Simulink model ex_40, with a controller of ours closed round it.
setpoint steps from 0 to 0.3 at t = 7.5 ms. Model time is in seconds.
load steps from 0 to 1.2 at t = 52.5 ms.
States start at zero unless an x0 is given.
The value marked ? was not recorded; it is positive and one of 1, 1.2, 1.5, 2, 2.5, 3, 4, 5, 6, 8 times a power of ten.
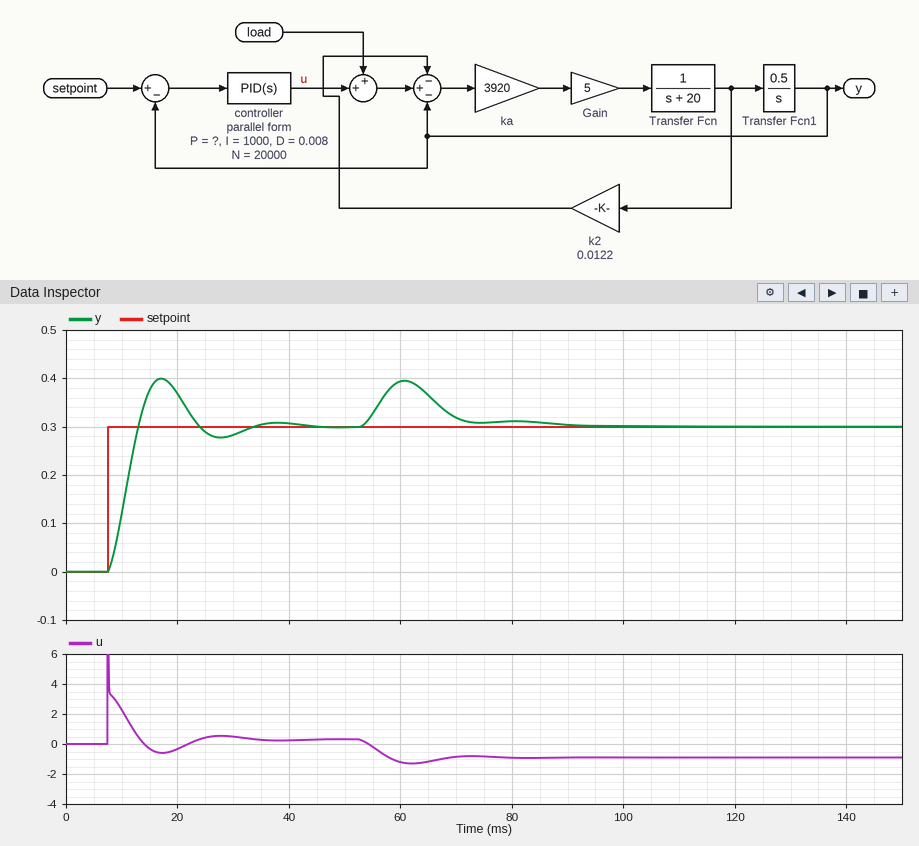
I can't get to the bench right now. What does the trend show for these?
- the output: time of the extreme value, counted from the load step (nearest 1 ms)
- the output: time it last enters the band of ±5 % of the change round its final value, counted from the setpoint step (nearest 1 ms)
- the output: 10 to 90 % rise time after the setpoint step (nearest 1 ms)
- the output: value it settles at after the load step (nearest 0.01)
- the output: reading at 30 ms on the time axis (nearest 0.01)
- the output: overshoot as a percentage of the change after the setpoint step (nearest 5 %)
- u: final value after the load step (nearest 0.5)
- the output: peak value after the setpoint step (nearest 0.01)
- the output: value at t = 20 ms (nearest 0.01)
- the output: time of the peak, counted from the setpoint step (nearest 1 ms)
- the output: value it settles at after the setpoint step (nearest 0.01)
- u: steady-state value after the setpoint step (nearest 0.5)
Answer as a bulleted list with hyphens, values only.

- 8 ms
- 23 ms
- 4 ms
- 0.30
- 0.28
- 35 %
- -1.0
- 0.40
- 0.37
- 10 ms
- 0.30
- 0.5
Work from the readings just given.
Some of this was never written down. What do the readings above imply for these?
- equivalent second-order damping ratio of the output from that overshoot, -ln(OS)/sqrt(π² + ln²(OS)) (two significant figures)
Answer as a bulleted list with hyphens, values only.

- 0.32
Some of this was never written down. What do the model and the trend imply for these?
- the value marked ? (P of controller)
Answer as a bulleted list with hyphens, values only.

- 12
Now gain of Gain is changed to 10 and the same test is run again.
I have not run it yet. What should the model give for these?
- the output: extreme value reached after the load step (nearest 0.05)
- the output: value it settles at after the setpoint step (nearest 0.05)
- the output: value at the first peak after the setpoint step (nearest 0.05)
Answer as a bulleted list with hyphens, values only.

- 0.40
- 0.30
- 0.35
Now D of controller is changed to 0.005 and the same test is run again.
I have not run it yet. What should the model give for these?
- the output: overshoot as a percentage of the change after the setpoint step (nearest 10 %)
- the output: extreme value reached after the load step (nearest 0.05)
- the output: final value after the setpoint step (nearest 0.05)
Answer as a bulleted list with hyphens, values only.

- 40 %
- 0.40
- 0.30
